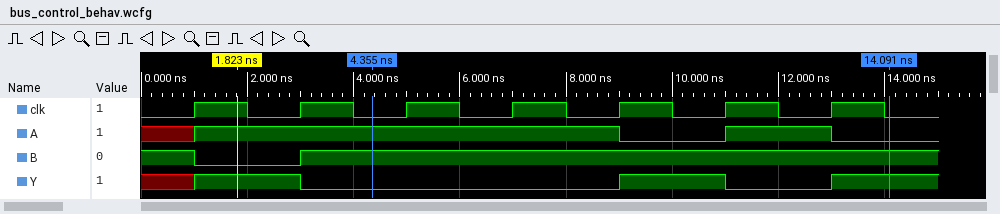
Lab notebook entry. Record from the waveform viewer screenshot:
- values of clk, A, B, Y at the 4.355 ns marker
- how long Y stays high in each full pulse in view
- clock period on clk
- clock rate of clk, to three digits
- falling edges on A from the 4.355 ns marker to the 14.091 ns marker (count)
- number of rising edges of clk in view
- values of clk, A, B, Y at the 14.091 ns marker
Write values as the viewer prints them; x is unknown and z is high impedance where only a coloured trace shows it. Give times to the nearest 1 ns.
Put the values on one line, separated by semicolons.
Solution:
clk=0, A=1, B=1, Y=0; 2 ns; 2 ns; 500 MHz; 2; 7; clk=0, A=0, B=1, Y=1
